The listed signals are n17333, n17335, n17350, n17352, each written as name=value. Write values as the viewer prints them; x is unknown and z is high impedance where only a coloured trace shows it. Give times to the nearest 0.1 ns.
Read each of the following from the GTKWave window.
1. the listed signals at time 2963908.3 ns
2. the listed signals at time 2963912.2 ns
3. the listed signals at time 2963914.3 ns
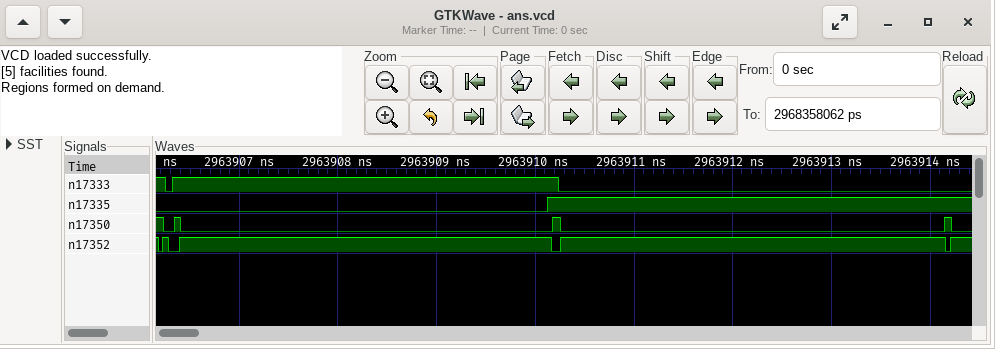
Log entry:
n17333=1, n17335=0, n17350=0, n17352=1
n17333=0, n17335=1, n17350=0, n17352=1
n17333=0, n17335=1, n17350=0, n17352=1
